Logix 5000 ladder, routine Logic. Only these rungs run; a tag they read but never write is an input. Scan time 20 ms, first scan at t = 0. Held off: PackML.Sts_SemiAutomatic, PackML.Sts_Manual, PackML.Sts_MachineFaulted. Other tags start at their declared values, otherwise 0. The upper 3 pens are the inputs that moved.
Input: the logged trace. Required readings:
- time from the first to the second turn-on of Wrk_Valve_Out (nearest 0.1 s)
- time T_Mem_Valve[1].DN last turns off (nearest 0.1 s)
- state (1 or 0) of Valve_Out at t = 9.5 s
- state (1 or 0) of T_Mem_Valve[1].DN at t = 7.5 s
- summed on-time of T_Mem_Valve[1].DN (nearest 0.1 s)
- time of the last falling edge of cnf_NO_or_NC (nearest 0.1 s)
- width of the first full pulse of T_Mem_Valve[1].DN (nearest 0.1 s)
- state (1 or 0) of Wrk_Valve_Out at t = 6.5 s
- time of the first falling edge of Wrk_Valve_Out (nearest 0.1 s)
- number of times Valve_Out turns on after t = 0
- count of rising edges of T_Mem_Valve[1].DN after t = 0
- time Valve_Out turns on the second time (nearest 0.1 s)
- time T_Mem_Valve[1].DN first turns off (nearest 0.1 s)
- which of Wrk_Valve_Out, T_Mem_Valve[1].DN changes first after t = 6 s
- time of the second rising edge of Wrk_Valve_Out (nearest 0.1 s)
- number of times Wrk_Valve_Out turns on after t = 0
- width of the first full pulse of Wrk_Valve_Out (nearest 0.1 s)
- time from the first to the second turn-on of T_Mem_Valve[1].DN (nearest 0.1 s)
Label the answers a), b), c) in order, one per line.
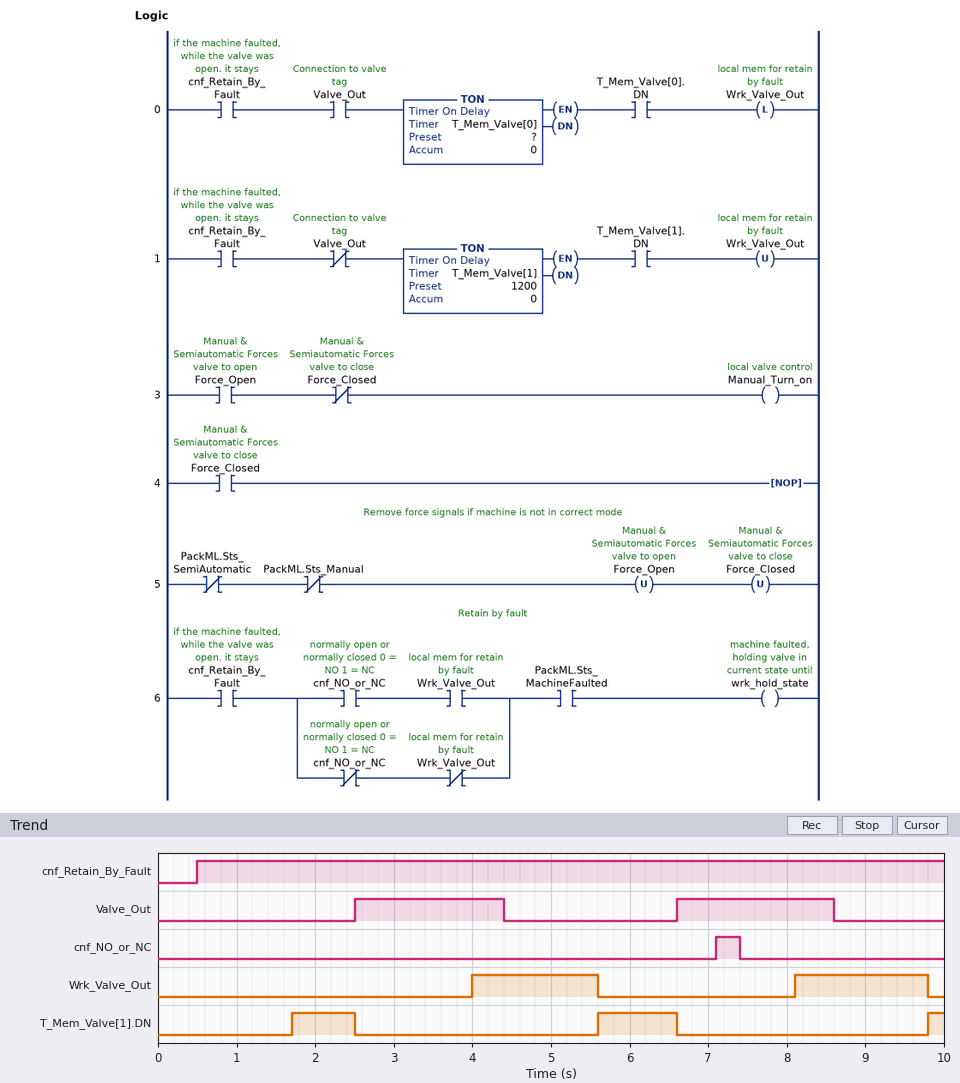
a) 4.1 s
b) 6.6 s
c) 0
d) 0
e) 2.0 s
f) 7.4 s
g) 0.8 s
h) 0
i) 5.6 s
j) 2
k) 3
l) 6.6 s
m) 2.5 s
n) T_Mem_Valve[1].DN
o) 8.1 s
p) 2
q) 1.6 s
r) 3.9 s
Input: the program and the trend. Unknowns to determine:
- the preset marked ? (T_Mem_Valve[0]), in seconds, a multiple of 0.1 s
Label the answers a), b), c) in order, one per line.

a) 1.5 s
